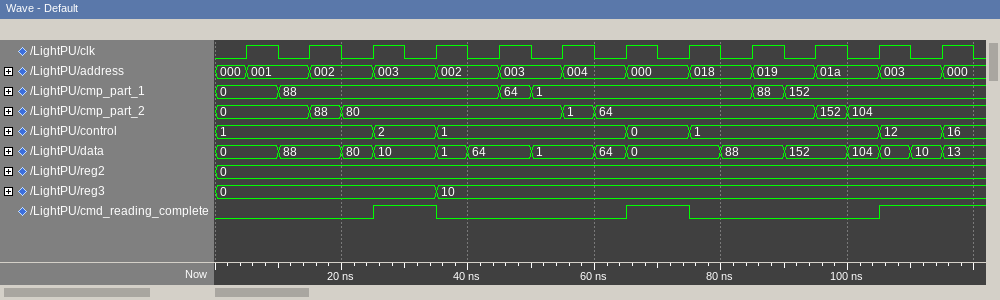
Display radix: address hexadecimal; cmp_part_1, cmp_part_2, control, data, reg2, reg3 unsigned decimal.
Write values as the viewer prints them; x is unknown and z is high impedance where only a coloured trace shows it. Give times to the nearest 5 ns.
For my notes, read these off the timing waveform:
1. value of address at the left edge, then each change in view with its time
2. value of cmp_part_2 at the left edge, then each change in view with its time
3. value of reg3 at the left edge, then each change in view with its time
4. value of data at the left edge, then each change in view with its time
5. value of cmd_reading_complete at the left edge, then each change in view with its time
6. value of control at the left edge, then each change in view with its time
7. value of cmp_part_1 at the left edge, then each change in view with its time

000, 001 at 5 ns, 002 at 15 ns, 003 at 25 ns, 002 at 35 ns, 003 at 45 ns, 004 at 55 ns, 000 at 65 ns, 018 at 75 ns, 019 at 85 ns, 01a at 95 ns, 003 at 105 ns, 000 at 115 ns
0, 88 at 15 ns, 80 at 20 ns, 1 at 55 ns, 64 at 60 ns, 152 at 95 ns, 104 at 100 ns
0, 10 at 35 ns
0, 88 at 10 ns, 80 at 20 ns, 10 at 25 ns, 1 at 35 ns, 64 at 40 ns, 1 at 50 ns, 64 at 60 ns, 0 at 65 ns, 88 at 80 ns, 152 at 90 ns, 104 at 100 ns, 0 at 105 ns, 10 at 110 ns, 13 at 115 ns
0, 1 at 25 ns, 0 at 35 ns, 1 at 65 ns, 0 at 75 ns, 1 at 105 ns
1, 2 at 25 ns, 1 at 35 ns, 0 at 65 ns, 1 at 75 ns, 12 at 105 ns, 16 at 115 ns
0, 88 at 10 ns, 64 at 45 ns, 1 at 50 ns, 88 at 85 ns, 152 at 90 ns
